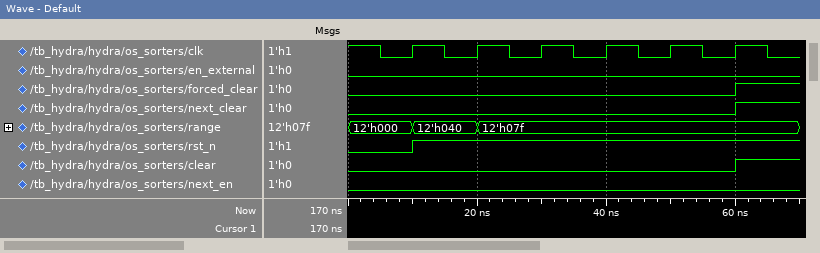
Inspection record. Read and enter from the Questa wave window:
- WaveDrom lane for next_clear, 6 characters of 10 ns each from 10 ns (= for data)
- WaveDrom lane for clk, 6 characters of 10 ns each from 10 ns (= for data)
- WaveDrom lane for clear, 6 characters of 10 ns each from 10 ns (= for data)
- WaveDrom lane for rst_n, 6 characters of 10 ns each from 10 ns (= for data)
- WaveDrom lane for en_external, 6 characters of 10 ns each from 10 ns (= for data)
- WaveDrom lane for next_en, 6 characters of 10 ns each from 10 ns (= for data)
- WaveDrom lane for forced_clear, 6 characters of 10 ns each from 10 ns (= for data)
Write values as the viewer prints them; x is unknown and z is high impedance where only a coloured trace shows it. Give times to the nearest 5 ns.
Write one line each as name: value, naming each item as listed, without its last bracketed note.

WaveDrom lane for next_clear, 6 characters of 10 ns each from 10 ns: {name: 'next_clear', wave: '0....1'}
WaveDrom lane for clk, 6 characters of 10 ns each from 10 ns: {name: 'clk', wave: 'p.....'}
WaveDrom lane for clear, 6 characters of 10 ns each from 10 ns: {name: 'clear', wave: '0....1'}
WaveDrom lane for rst_n, 6 characters of 10 ns each from 10 ns: {name: 'rst_n', wave: '1.....'}
WaveDrom lane for en_external, 6 characters of 10 ns each from 10 ns: {name: 'en_external', wave: '0.....'}
WaveDrom lane for next_en, 6 characters of 10 ns each from 10 ns: {name: 'next_en', wave: '0.....'}
WaveDrom lane for forced_clear, 6 characters of 10 ns each from 10 ns: {name: 'forced_clear', wave: '0....1'}
